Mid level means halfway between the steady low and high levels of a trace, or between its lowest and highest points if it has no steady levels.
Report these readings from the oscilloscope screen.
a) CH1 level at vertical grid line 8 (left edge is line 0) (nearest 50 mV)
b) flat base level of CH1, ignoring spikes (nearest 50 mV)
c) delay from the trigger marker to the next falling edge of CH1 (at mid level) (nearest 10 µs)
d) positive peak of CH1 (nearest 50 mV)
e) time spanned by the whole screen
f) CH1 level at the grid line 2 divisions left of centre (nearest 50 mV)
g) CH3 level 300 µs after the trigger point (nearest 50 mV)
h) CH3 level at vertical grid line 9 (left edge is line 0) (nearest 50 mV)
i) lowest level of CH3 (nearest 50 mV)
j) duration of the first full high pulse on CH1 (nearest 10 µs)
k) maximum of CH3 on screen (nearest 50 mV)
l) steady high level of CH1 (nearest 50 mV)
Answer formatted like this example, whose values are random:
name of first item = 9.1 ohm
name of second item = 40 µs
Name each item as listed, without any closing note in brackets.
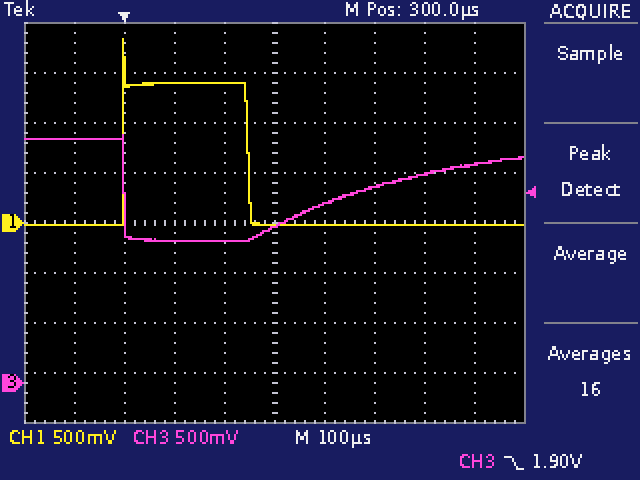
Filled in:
CH1 level at vertical grid line 8 (left edge is line 0) = 0 mV
flat base level of CH1, ignoring spikes = 0 mV
delay from the trigger marker to the next falling edge of CH1 (at mid level) = 250 µs
positive peak of CH1 = 1.85 V
time spanned by the whole screen = 1 ms
CH1 level at the grid line 2 divisions left of centre = 1.40 V
CH3 level 300 µs after the trigger point = 1.55 V
CH3 level at vertical grid line 9 (left edge is line 0) = 2.20 V
lowest level of CH3 = 1.40 V
duration of the first full high pulse on CH1 = 250 µs
maximum of CH3 on screen = 2.50 V
steady high level of CH1 = 1.40 V
